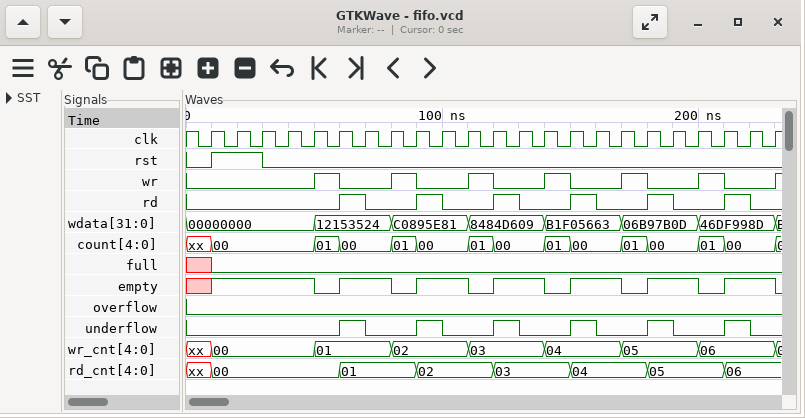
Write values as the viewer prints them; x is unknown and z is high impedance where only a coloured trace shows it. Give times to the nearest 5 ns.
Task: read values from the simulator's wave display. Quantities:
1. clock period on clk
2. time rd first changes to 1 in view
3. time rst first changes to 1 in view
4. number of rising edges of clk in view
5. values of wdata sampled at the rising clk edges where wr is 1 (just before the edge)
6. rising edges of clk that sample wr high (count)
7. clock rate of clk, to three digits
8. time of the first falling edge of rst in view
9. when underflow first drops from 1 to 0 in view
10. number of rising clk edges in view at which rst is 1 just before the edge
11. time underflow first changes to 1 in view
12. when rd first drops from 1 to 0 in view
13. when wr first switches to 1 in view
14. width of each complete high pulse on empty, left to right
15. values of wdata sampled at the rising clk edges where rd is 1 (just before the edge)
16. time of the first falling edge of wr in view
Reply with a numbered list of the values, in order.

1. 10 ns
2. 60 ns
3. 10 ns
4. 23
5. 12153524, C0895E81, 8484D609, B1F05663, 06B97B0D, 46DF998D
6. 6
7. 100 MHz
8. 30 ns
9. 70 ns
10. 2
11. 60 ns
12. 70 ns
13. 50 ns
14. 20 ns, 20 ns, 20 ns, 20 ns, 20 ns, 20 ns
15. 12153524, C0895E81, 8484D609, B1F05663, 06B97B0D, 46DF998D
16. 60 ns
